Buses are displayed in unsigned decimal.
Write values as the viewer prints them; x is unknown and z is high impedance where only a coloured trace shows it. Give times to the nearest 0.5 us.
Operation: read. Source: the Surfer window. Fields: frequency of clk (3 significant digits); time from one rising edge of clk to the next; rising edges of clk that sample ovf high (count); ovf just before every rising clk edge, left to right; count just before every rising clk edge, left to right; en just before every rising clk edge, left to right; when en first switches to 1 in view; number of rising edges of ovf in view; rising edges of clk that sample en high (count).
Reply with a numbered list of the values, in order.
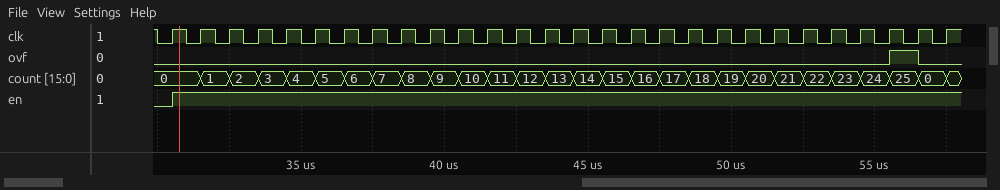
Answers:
1. 1.00 MHz
2. 1 us
3. 1
4. 0 0 0 0 0 0 0 0 0 0 0 0 0 0 0 0 0 0 0 0 0 0 0 0 0 0 1 0
5. 0, 0, 1, 2, 3, 4, 5, 6, 7, 8, 9, 10, 11, 12, 13, 14, 15, 16, 17, 18, 19, 20, 21, 22, 23, 24, 25, 0
6. 0 1 1 1 1 1 1 1 1 1 1 1 1 1 1 1 1 1 1 1 1 1 1 1 1 1 1 1
7. 30.5 us
8. 1
9. 27
